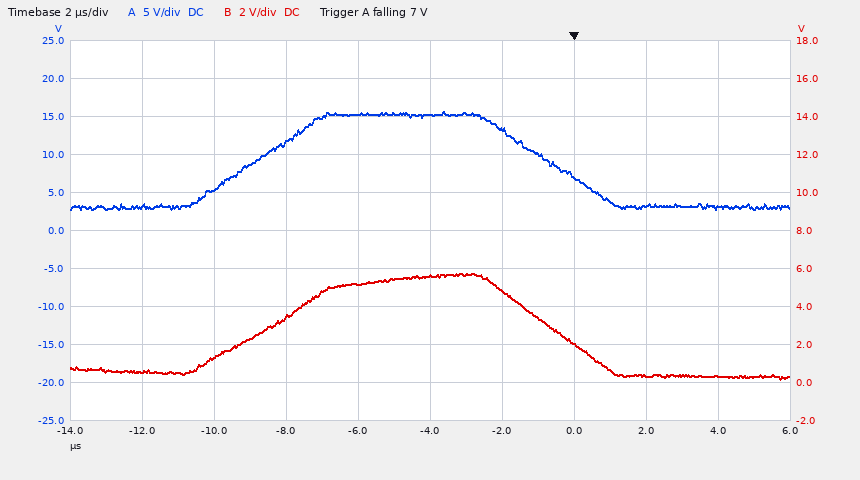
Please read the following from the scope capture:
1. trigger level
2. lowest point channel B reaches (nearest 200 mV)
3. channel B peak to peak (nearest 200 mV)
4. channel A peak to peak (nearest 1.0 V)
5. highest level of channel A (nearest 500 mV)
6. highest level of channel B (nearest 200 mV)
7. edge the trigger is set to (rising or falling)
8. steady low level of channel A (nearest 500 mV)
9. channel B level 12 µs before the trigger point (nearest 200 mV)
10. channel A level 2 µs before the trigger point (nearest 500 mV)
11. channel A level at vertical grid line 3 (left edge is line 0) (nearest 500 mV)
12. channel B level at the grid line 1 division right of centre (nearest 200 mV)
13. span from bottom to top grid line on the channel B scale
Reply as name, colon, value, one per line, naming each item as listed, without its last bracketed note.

trigger level: 7 V
lowest point channel B reaches: 200 mV
channel B peak to peak: 5.6 V
channel A peak to peak: 13.0 V
highest level of channel A: 15.5 V
highest level of channel B: 5.8 V
edge the trigger is set to: falling
steady low level of channel A: 3.0 V
channel B level 12 µs before the trigger point: 600 mV
channel A level 2 µs before the trigger point: 13.5 V
channel A level at vertical grid line 3 (left edge is line 0): 11.5 V
channel B level at the grid line 1 division right of centre: 4.8 V
span from bottom to top grid line on the channel B scale: 20 V
